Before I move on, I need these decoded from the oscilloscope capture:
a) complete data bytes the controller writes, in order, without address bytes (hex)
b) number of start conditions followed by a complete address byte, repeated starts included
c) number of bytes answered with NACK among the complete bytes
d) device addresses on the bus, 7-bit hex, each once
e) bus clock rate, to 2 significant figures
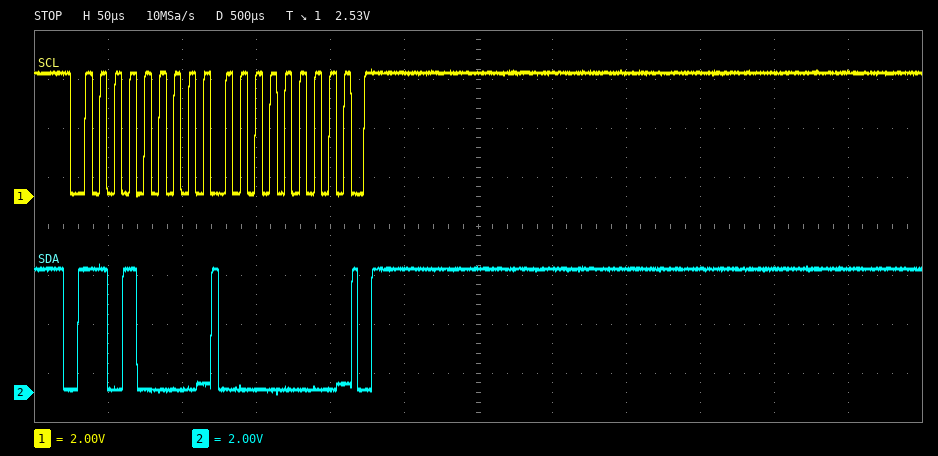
00
1
0
0x68
100 kHz
